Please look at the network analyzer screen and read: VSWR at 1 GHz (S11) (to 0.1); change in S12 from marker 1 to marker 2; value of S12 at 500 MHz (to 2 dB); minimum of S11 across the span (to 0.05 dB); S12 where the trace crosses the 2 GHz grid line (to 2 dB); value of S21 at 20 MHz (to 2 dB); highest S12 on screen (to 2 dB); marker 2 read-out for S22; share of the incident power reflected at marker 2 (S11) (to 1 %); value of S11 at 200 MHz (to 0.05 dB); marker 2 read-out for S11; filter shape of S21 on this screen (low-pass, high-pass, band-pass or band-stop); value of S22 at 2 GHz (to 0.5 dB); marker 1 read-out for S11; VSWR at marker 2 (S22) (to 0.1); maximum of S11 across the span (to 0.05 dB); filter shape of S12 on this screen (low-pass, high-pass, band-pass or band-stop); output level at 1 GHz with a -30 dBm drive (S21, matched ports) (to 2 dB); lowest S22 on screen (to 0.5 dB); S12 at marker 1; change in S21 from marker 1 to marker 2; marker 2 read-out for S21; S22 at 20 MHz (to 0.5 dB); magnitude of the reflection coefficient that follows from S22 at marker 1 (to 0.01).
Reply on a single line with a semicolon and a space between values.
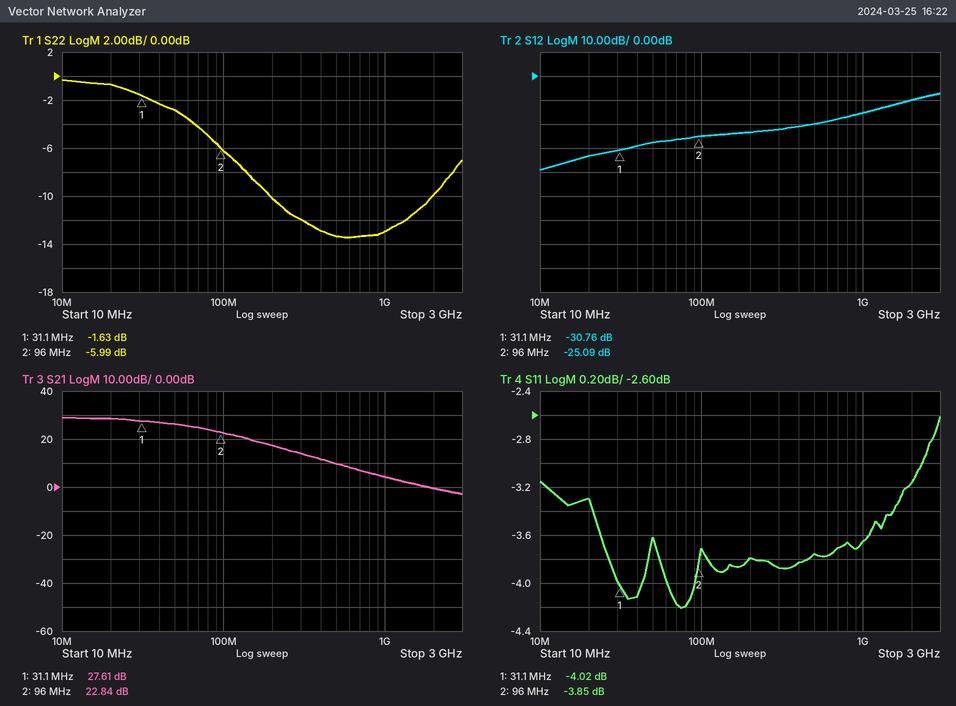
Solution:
4.8; 5.67 dB; -20 dB; -4.20 dB; -10 dB; 28 dB; -8 dB; -5.99 dB; 41 %; -3.80 dB; -3.85 dB; low-pass; -10.0 dB; -4.02 dB; 3.0; -2.60 dB; high-pass; -26 dBm; -13.5 dB; -30.76 dB; -4.77 dB; 22.84 dB; -0.5 dB; 0.83
